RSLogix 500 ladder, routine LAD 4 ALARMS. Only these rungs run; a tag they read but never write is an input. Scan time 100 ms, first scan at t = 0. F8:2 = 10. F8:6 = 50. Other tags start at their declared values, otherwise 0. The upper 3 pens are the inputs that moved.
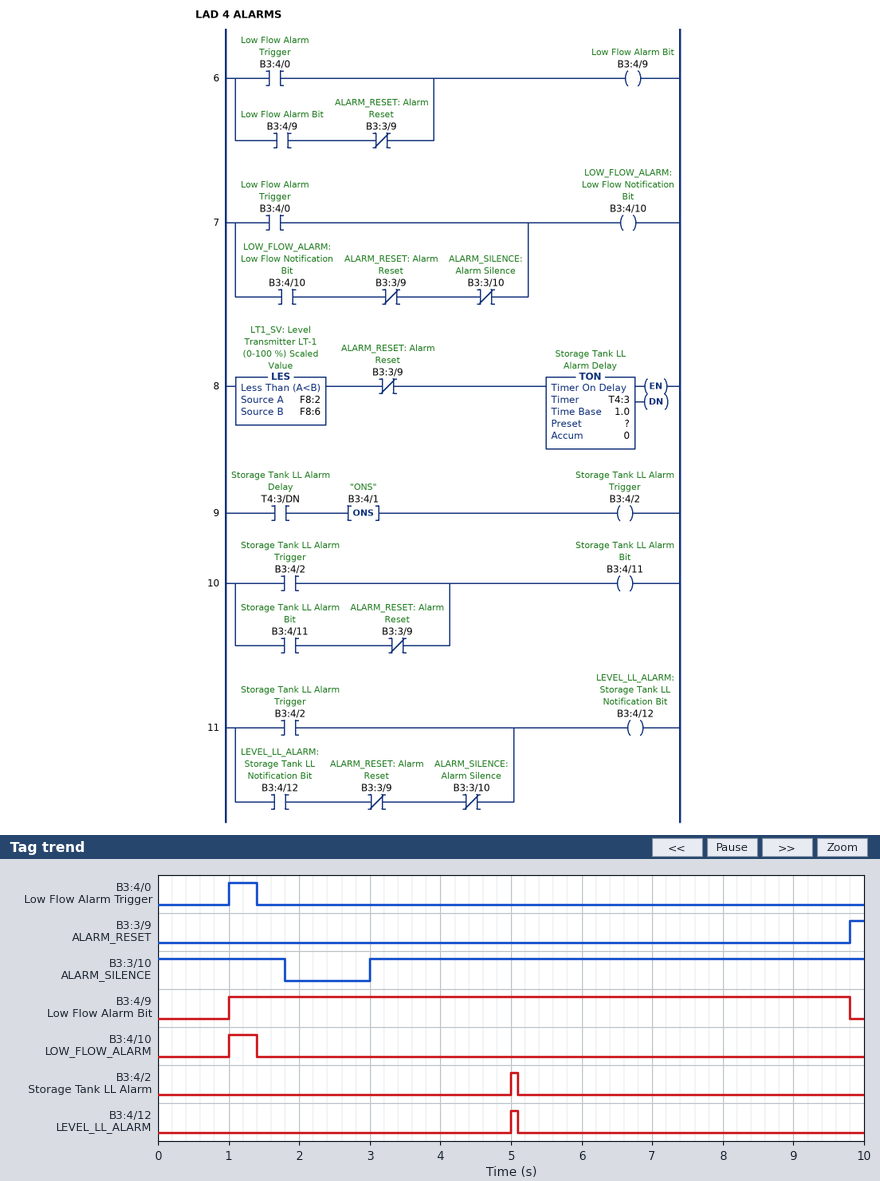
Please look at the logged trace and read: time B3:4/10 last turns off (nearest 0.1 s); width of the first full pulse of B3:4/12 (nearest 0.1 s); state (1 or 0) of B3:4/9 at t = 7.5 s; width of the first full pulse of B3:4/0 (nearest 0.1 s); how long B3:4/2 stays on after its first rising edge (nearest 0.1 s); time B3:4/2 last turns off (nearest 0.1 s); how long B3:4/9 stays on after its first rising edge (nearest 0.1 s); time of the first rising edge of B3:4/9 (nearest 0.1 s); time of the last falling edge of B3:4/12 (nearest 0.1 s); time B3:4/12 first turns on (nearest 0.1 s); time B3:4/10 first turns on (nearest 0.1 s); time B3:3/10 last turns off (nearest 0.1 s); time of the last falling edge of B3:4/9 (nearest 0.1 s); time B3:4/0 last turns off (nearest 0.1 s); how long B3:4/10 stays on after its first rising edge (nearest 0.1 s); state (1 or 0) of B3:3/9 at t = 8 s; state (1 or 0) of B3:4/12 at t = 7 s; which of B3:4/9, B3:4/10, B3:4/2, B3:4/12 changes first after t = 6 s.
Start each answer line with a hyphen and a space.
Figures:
- 1.4 s
- 0.1 s
- 1
- 0.4 s
- 0.1 s
- 5.1 s
- 8.8 s
- 1.0 s
- 5.1 s
- 5.0 s
- 1.0 s
- 1.8 s
- 9.8 s
- 1.4 s
- 0.4 s
- 0
- 0
- B3:4/9
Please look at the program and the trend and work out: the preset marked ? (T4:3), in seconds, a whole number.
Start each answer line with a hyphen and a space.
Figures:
- 5 s
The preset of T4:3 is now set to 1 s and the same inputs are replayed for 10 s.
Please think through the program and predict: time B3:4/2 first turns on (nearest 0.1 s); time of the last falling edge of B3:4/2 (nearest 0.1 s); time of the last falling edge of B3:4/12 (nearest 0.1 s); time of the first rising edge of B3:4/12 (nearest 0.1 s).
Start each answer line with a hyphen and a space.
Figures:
- 1.0 s
- 1.1 s
- 1.1 s
- 1.0 s
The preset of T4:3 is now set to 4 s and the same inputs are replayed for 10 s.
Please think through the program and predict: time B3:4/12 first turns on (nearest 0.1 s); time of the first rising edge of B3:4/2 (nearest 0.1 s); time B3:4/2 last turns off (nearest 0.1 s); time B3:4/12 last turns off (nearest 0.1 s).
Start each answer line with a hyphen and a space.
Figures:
- 4.0 s
- 4.0 s
- 4.1 s
- 4.1 s
